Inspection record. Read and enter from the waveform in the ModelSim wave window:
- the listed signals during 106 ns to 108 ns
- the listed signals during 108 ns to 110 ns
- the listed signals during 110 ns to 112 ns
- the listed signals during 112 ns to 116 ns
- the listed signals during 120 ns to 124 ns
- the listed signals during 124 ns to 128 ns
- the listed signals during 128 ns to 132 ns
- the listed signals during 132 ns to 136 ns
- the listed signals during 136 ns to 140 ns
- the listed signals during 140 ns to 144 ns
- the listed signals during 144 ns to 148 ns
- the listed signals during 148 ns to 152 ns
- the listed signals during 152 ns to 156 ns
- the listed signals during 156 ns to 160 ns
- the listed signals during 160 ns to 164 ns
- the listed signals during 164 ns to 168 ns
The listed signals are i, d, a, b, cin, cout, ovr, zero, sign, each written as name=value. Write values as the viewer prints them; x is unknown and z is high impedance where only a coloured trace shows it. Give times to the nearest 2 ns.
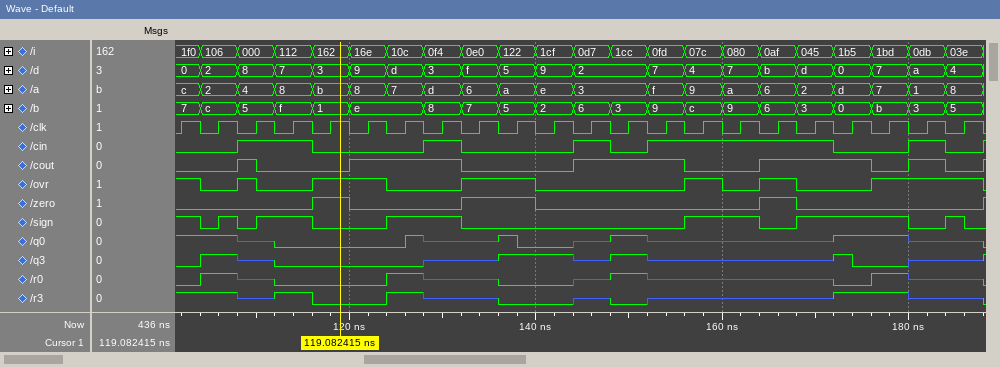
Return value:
i=106, d=2, a=2, b=c, cin=0, cout=0, ovr=0, zero=0, sign=1
i=000, d=8, a=4, b=5, cin=1, cout=1, ovr=1, zero=0, sign=0
i=000, d=8, a=4, b=5, cin=1, cout=0, ovr=0, zero=0, sign=1
i=112, d=7, a=8, b=f, cin=1, cout=0, ovr=0, zero=0, sign=1
i=16e, d=9, a=8, b=e, cin=0, cout=1, ovr=1, zero=0, sign=0
i=10c, d=d, a=7, b=e, cin=0, cout=1, ovr=0, zero=0, sign=1
i=0f4, d=3, a=d, b=8, cin=1, cout=1, ovr=0, zero=0, sign=1
i=0e0, d=f, a=6, b=7, cin=0, cout=0, ovr=1, zero=1, sign=0
i=122, d=5, a=a, b=5, cin=0, cout=0, ovr=1, zero=1, sign=0
i=1cf, d=9, a=e, b=2, cin=0, cout=0, ovr=0, zero=0, sign=0
i=0d7, d=2, a=3, b=6, cin=1, cout=1, ovr=0, zero=0, sign=0
i=1cc, d=2, a=3, b=3, cin=0, cout=1, ovr=0, zero=0, sign=0
i=0fd, d=7, a=f, b=9, cin=1, cout=1, ovr=0, zero=0, sign=0
i=07c, d=4, a=9, b=c, cin=1, cout=0, ovr=1, zero=0, sign=1
i=080, d=7, a=a, b=9, cin=1, cout=0, ovr=0, zero=0, sign=1
i=0af, d=b, a=6, b=6, cin=1, cout=1, ovr=1, zero=1, sign=0
